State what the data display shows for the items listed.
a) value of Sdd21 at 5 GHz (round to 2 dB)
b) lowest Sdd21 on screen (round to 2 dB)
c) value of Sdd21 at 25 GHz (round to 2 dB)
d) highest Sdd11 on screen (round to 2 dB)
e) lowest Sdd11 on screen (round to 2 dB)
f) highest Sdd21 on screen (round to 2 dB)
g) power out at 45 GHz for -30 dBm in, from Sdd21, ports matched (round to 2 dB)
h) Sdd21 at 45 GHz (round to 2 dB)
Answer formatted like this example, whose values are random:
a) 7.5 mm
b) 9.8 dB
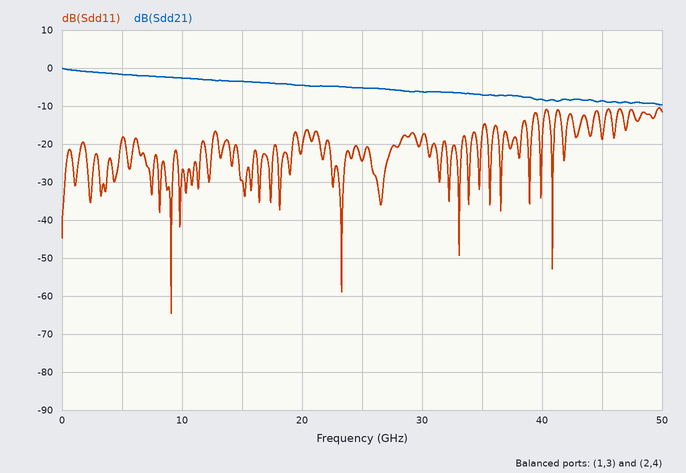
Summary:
a) -2 dB
b) -10 dB
c) -6 dB
d) -10 dB
e) -64 dB
f) 0 dB
g) -38 dBm
h) -8 dB
